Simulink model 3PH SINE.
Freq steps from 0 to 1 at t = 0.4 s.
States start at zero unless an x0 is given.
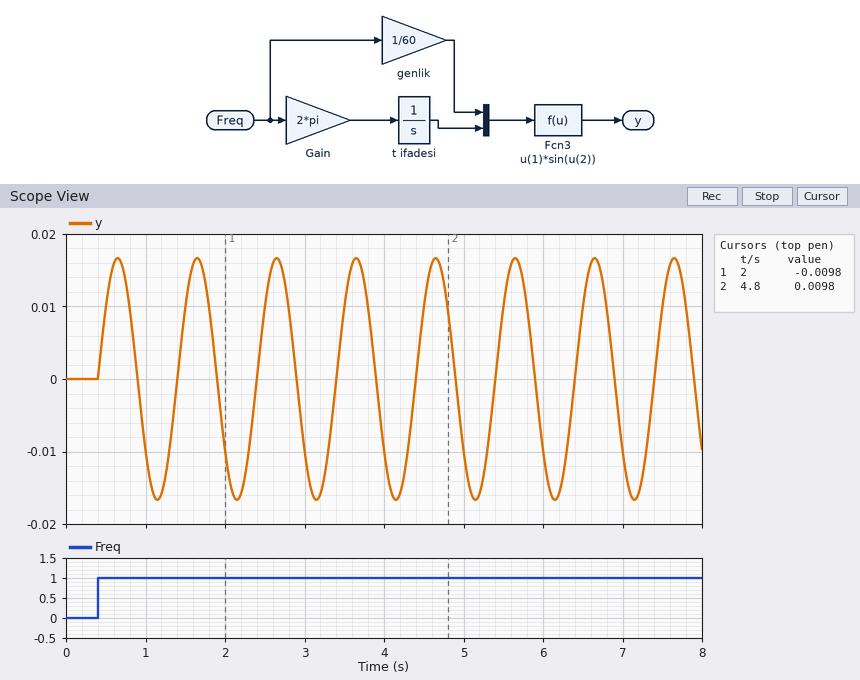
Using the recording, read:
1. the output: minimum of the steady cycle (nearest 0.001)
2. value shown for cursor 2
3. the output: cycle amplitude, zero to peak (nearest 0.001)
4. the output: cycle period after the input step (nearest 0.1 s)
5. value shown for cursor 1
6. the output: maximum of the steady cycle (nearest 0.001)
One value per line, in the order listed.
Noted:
-0.017
0.0098
0.017
1.0 s
-0.0098
0.017
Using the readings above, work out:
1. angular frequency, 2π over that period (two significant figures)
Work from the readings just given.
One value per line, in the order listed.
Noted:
6.3 rad/s
